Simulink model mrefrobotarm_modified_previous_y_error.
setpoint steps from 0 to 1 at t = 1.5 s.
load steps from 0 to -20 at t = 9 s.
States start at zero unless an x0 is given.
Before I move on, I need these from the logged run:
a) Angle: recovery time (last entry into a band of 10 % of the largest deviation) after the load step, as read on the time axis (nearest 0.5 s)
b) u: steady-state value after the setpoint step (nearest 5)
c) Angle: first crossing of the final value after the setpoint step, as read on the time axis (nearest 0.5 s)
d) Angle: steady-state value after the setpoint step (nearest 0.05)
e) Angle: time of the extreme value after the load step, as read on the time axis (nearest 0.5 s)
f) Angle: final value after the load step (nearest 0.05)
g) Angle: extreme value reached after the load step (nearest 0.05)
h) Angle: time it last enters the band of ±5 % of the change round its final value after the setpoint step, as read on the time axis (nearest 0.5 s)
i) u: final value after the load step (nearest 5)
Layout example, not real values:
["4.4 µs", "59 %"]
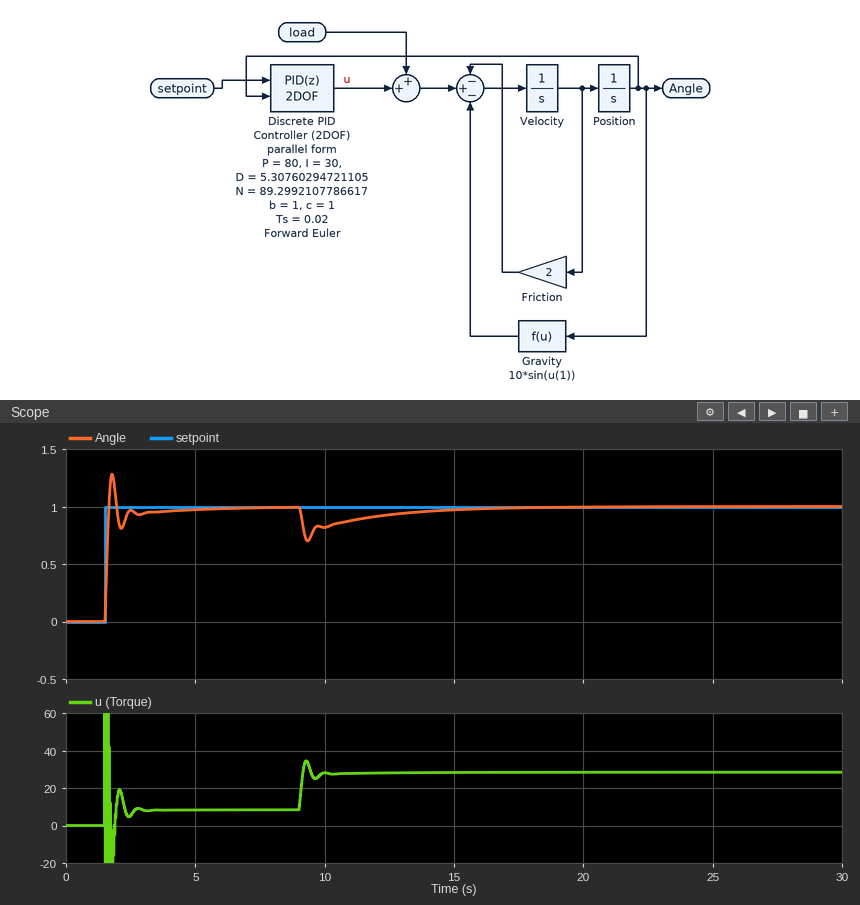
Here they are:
["15.0 s", "10", "1.5 s", "1.00", "9.5 s", "1.00", "0.70", "3.0 s", "30"]
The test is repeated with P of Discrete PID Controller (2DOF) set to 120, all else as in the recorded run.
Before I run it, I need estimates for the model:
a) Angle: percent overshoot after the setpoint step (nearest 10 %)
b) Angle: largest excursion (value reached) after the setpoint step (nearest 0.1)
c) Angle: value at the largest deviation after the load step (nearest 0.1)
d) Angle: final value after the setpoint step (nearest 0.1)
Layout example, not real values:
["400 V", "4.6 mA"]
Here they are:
["40 %", "1.4", "0.8", "1.0"]
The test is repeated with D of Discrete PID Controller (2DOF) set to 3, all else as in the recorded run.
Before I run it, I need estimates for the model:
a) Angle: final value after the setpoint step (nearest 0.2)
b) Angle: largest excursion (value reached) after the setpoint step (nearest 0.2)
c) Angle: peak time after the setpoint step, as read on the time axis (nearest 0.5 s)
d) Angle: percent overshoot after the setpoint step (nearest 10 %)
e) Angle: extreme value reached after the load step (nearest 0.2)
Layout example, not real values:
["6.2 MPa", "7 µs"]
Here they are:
["1.0", "1.4", "2.0 s", "40 %", "0.6"]
